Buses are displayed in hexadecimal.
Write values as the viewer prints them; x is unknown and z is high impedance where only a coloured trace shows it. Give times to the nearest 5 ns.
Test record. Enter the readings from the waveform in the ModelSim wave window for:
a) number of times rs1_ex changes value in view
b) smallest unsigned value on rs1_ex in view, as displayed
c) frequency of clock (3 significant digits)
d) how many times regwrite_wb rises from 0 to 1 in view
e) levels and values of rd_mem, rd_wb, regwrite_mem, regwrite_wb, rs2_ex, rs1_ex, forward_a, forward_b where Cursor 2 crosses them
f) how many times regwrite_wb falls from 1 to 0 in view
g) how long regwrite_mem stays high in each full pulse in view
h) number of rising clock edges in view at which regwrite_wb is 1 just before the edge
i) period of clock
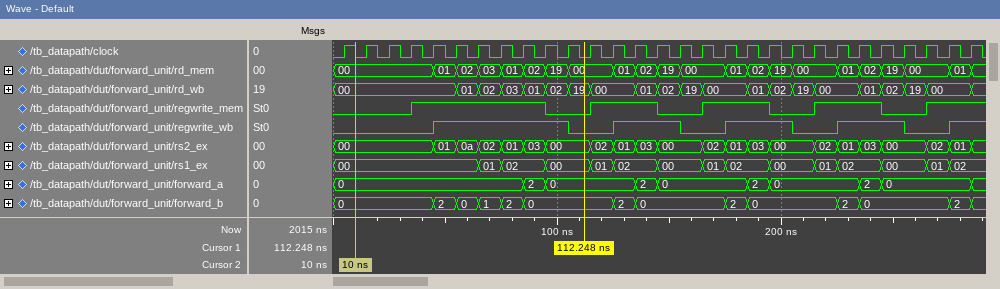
14
00
100 MHz
5
rd_mem=00, rd_wb=00, regwrite_mem=0, regwrite_wb=0, rs2_ex=00, rs1_ex=00, forward_a=0, forward_b=0
4
60 ns, 30 ns, 30 ns, 30 ns
16
10 ns
